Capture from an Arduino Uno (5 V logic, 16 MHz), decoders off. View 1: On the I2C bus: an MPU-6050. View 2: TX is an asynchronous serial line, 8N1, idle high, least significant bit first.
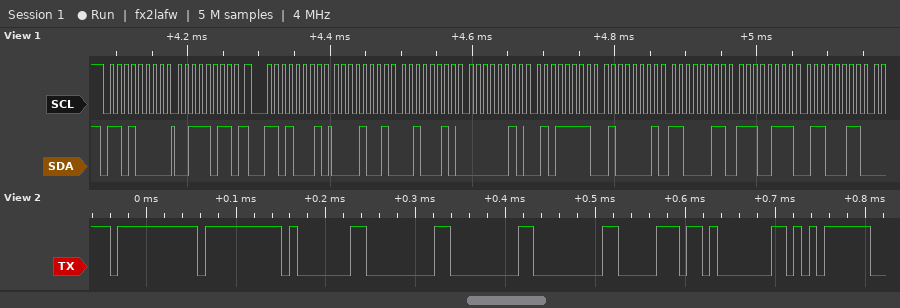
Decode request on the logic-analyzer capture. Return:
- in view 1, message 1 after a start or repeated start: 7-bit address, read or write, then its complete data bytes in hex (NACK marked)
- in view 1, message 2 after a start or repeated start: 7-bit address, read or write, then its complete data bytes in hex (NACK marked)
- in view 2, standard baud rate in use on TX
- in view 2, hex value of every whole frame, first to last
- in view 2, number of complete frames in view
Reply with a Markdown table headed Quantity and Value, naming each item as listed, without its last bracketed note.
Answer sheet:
| Quantity | Value |
|---|---|
| in view 1, message 1 after a start or repeated start: 7-bit address, read or write, then its complete data bytes in hex | 0x68 write: 3B |
| in view 1, message 2 after a start or repeated start: 7-bit address, read or write, then its complete data bytes in hex | 0x68 read: 09 22 02 5F 41 C3 E7 63 |
| in view 2, standard baud rate in use on TX | 115200 baud |
| in view 2, hex value of every whole frame, first to last | FF FF 01 00 00 00 70 01 F5 |
| in view 2, number of complete frames in view | 9 |
